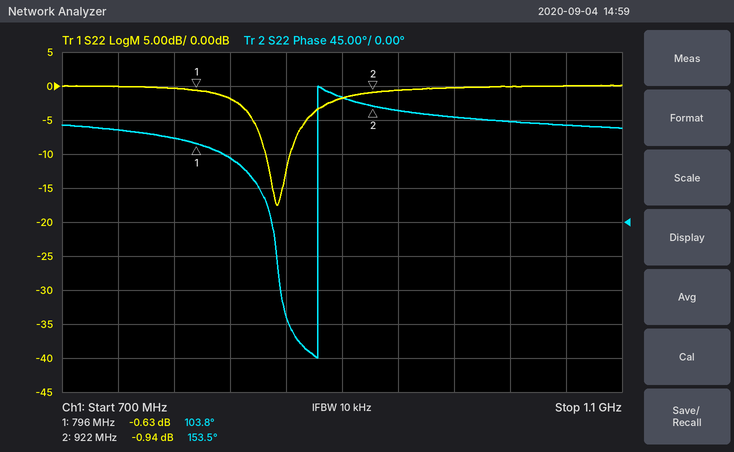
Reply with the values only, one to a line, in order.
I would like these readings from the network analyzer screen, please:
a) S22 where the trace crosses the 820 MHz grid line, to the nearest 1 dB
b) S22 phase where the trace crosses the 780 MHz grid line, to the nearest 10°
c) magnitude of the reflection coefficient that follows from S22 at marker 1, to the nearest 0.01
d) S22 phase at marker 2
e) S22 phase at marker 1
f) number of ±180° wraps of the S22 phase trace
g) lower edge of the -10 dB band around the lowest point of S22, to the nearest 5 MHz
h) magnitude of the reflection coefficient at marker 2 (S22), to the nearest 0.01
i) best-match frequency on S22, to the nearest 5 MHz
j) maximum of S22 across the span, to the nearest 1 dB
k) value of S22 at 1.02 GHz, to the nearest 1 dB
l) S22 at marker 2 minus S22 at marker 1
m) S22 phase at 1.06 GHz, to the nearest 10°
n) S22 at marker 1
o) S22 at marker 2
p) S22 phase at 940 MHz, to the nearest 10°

-2 dB
110°
0.93
153.5°
103.8°
1
845 MHz
0.90
855 MHz
0 dB
0 dB
-0.31 dB
130°
-0.63 dB
-0.94 dB
150°
